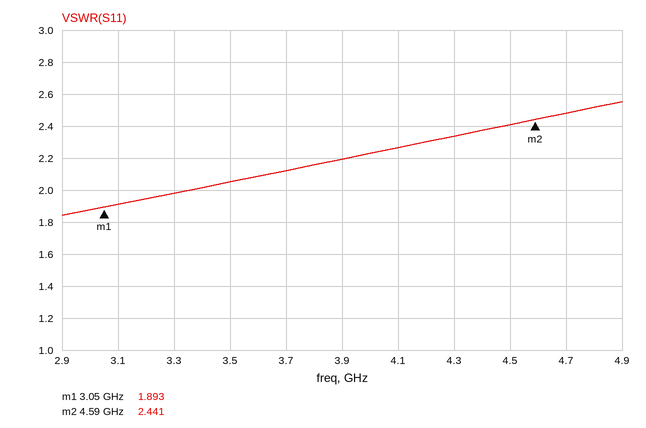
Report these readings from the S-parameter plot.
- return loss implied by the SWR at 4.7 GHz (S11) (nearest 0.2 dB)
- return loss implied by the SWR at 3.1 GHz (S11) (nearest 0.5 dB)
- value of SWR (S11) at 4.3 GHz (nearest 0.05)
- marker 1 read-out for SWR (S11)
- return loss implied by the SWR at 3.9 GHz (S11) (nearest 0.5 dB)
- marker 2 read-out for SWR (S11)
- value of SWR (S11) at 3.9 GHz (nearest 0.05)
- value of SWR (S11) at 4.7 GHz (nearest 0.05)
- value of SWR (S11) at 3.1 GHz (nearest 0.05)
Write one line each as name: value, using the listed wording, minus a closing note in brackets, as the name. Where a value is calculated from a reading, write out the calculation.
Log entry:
return loss implied by the SWR at 4.7 GHz (S11): −20 log10((2.5 − 1)/(2.5 + 1)) ≈ 7.4 dB
return loss implied by the SWR at 3.1 GHz (S11): −20 log10((1.9 − 1)/(1.9 + 1)) ≈ 10.2 dB, so 10.0 dB to the nearest 0.5 dB
value of SWR (S11) at 4.3 GHz: 2.35
marker 1 read-out for SWR: 1.893
return loss implied by the SWR at 3.9 GHz (S11): −20 log10((2.2 − 1)/(2.2 + 1)) ≈ 8.5 dB
marker 2 read-out for SWR: 2.441
value of SWR (S11) at 3.9 GHz: 2.20
value of SWR (S11) at 4.7 GHz: 2.50
value of SWR (S11) at 3.1 GHz: 1.90
